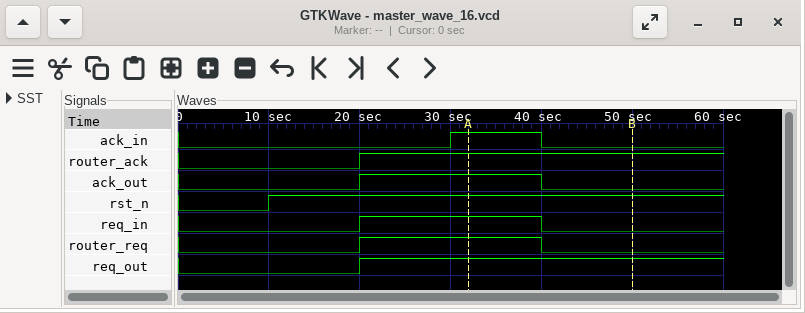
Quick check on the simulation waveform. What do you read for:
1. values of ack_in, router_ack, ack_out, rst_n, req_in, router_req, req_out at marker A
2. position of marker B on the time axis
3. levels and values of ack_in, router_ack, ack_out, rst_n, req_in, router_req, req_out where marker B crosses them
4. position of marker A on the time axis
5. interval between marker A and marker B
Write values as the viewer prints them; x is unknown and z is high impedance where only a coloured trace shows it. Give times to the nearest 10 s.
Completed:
ack_in=1, router_ack=1, ack_out=1, rst_n=1, req_in=1, router_req=1, req_out=1
50 s
ack_in=0, router_ack=1, ack_out=0, rst_n=1, req_in=0, router_req=0, req_out=1
30 s
20 s
